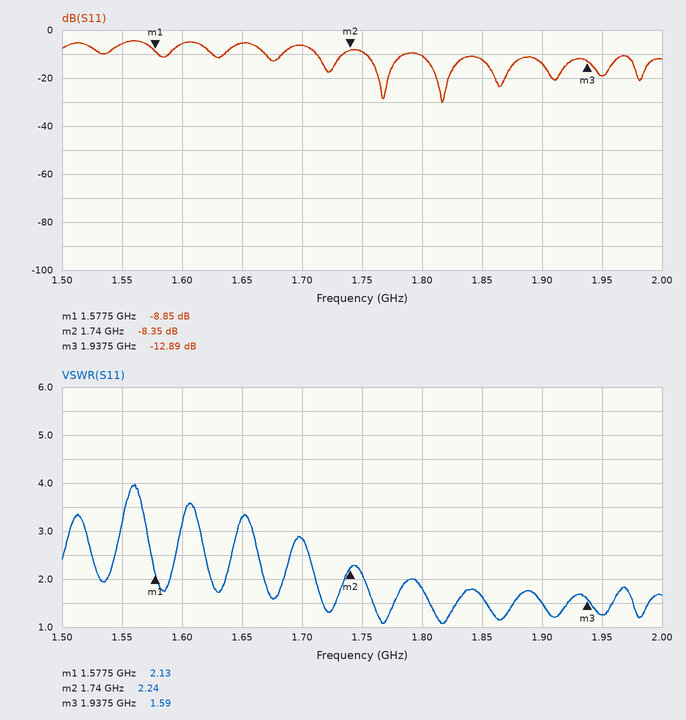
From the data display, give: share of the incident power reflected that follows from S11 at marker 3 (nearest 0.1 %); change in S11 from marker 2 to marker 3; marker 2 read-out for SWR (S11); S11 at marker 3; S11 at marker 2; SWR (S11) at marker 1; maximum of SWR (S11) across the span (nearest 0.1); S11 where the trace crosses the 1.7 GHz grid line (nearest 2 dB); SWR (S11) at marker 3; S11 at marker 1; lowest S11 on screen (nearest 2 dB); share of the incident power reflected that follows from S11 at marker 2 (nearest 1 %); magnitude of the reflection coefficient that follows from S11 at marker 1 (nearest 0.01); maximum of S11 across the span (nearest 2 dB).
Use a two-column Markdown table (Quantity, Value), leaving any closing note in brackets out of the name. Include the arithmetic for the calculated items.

| Quantity | Value |
|---|---|
| share of the incident power reflected that follows from S11 at marker 3 | 10^(-12.89/10) ≈ 5.1 % |
| change in S11 from marker 2 to marker 3 | -12.89 − (-8.35) = -4.54 dB |
| marker 2 read-out for SWR | 2.24 |
| S11 at marker 3 | -12.89 dB |
| S11 at marker 2 | -8.35 dB |
| SWR (S11) at marker 1 | 2.13 |
| maximum of SWR (S11) across the span | 4.0 |
| S11 where the trace crosses the 1.7 GHz grid line | -6 dB |
| SWR (S11) at marker 3 | 1.59 |
| S11 at marker 1 | -8.85 dB |
| lowest S11 on screen | -30 dB |
| share of the incident power reflected that follows from S11 at marker 2 | 10^(-8.35/10) ≈ 15 % |
| magnitude of the reflection coefficient that follows from S11 at marker 1 | 10^(-8.85/20) ≈ 0.36 |
| maximum of S11 across the span | -4 dB |
